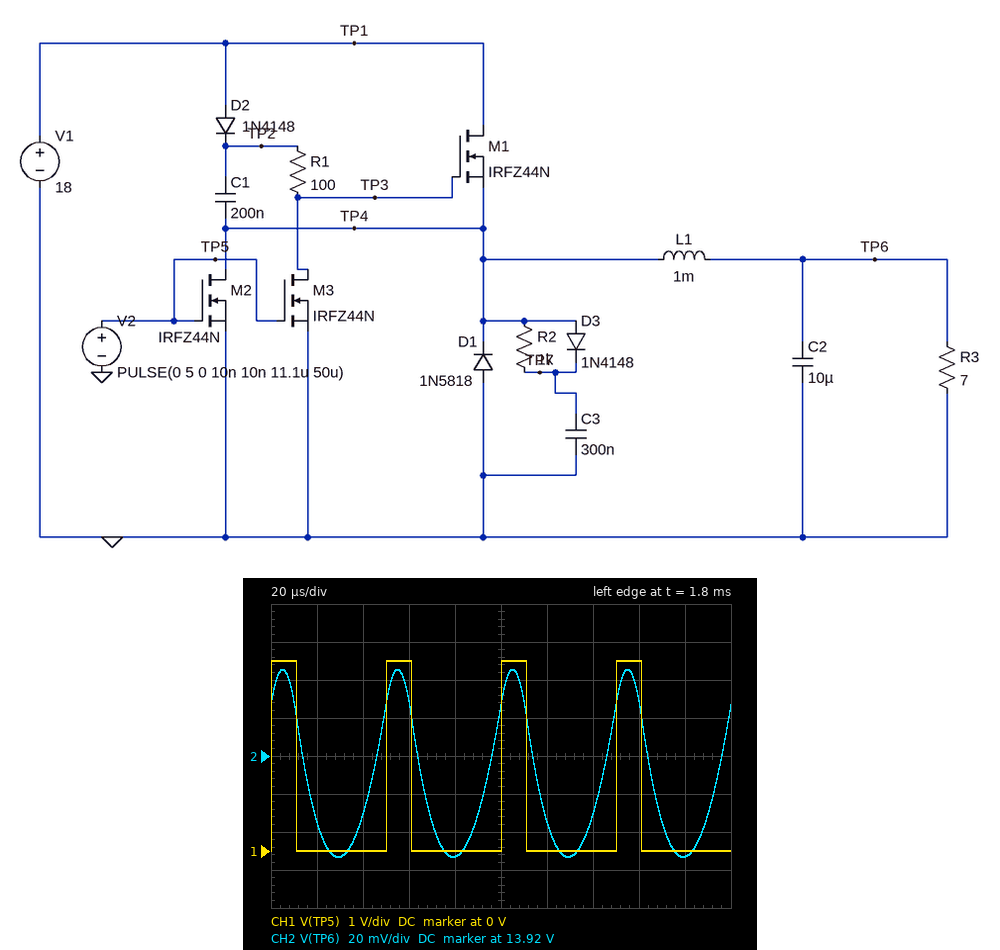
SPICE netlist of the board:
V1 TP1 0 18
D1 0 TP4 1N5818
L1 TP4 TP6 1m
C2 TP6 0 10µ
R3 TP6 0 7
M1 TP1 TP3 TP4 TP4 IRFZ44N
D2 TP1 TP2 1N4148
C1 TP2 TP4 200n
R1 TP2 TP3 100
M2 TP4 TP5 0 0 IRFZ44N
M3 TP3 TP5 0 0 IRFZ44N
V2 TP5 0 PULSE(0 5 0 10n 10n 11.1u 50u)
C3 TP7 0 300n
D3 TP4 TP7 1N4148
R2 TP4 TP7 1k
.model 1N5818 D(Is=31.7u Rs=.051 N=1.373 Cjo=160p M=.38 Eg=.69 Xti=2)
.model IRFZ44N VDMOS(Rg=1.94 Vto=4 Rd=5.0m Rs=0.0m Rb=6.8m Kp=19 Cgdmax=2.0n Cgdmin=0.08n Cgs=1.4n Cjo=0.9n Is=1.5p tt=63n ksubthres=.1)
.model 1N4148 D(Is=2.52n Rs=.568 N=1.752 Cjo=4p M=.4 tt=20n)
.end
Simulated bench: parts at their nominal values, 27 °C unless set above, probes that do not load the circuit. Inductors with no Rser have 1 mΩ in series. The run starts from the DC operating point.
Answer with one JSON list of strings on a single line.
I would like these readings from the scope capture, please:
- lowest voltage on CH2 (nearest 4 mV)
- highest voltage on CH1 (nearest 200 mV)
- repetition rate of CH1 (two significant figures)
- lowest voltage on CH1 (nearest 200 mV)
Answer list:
["13.868 V", "5.0 V", "20 kHz", "0 V"]
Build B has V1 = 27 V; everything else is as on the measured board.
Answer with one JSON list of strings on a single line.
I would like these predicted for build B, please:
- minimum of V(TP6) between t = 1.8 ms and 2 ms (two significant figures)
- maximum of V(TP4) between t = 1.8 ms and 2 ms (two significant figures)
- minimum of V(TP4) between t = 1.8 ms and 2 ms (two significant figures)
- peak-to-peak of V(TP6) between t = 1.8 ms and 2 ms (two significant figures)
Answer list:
["21 V", "27 V", "-560 mV", "150 mV"]
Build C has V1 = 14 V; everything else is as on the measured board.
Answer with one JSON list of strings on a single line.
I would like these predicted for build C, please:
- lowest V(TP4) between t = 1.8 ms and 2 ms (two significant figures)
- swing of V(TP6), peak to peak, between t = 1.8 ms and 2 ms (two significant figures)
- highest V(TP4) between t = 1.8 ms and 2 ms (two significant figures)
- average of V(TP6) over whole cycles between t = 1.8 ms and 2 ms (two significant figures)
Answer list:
["-470 mV", "77 mV", "14 V", "11 V"]
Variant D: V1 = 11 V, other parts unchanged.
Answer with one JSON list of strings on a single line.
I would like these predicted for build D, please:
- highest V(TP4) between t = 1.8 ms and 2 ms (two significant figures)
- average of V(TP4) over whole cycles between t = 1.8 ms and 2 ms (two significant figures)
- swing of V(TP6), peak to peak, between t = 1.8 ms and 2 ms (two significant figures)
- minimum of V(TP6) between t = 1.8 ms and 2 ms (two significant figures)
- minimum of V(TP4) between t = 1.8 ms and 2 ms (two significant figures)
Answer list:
["11 V", "8.5 V", "61 mV", "8.4 V", "-450 mV"]
